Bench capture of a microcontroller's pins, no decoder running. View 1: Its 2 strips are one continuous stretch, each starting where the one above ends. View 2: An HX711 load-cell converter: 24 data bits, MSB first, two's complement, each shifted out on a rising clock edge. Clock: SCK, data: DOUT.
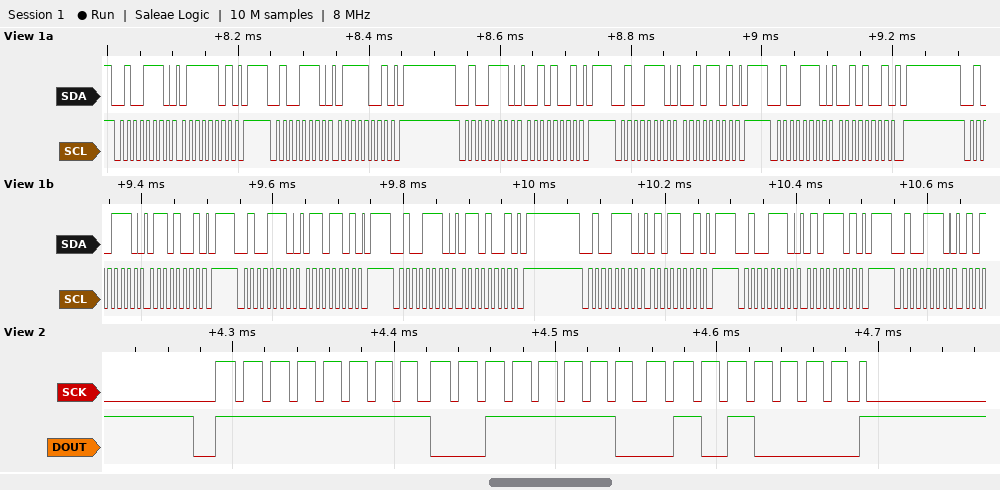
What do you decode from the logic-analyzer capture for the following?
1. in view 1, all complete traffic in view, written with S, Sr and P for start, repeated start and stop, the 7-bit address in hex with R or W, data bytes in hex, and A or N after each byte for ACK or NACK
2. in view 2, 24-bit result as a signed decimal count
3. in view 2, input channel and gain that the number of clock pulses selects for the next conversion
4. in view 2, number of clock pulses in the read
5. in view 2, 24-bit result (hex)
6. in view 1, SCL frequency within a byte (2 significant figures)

S 27W A 7D A P S 27W A 79 A P S 27W A 29 A P S 27W A 2D A P S 27W A 29 A P S 27W A 69 A P S 27W A 6D A P S 27W A 69 A P S 27W A 59 A P S 27W A 5D A P S 27W A
-49584
channel A, gain 128
25
0xFF3E50
100 kHz
